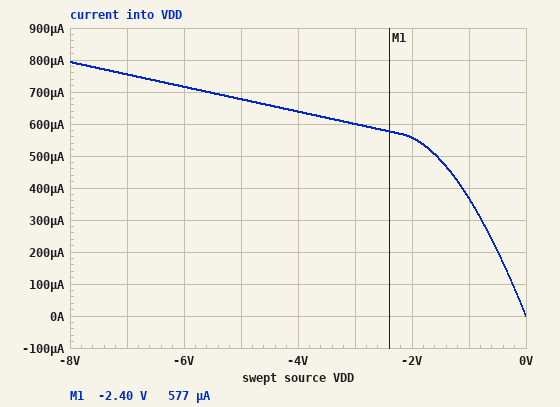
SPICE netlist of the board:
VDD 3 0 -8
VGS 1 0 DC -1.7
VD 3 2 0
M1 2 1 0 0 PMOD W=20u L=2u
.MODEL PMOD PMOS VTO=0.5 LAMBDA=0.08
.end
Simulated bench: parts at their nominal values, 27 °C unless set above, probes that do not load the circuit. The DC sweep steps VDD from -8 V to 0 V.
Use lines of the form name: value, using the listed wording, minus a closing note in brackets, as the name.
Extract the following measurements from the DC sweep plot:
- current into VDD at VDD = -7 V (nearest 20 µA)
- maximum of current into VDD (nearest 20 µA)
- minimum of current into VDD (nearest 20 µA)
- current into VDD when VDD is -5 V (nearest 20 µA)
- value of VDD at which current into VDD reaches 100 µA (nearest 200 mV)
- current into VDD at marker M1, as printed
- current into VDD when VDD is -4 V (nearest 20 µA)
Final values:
current into VDD at VDD = -7 V: 760 µA
maximum of current into VDD: 800 µA
minimum of current into VDD: 0 A
current into VDD when VDD is -5 V: 680 µA
value of VDD at which current into VDD reaches 100 µA: -200 mV
current into VDD at marker M1, as printed: 577 µA
current into VDD when VDD is -4 V: 640 µA
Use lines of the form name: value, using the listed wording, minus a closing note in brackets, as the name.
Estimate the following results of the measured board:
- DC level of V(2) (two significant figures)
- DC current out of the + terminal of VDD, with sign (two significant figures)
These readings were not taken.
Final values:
DC level of V(2): -8.0 V
DC current out of the + terminal of VDD, with sign: -790 µA
